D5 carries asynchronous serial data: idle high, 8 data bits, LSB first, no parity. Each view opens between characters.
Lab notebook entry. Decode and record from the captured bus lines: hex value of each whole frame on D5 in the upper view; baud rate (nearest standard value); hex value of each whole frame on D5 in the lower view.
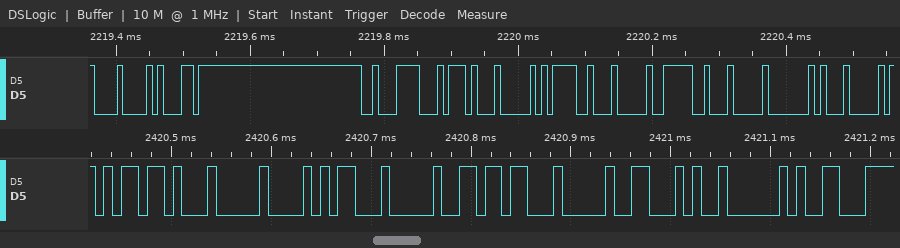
08, B1, E2, 74, 04, 3D, 04, 3E, 04, 40, 04
115200 baud
6D, 04, A8, 04, B6, 04, 46, 02, 19
